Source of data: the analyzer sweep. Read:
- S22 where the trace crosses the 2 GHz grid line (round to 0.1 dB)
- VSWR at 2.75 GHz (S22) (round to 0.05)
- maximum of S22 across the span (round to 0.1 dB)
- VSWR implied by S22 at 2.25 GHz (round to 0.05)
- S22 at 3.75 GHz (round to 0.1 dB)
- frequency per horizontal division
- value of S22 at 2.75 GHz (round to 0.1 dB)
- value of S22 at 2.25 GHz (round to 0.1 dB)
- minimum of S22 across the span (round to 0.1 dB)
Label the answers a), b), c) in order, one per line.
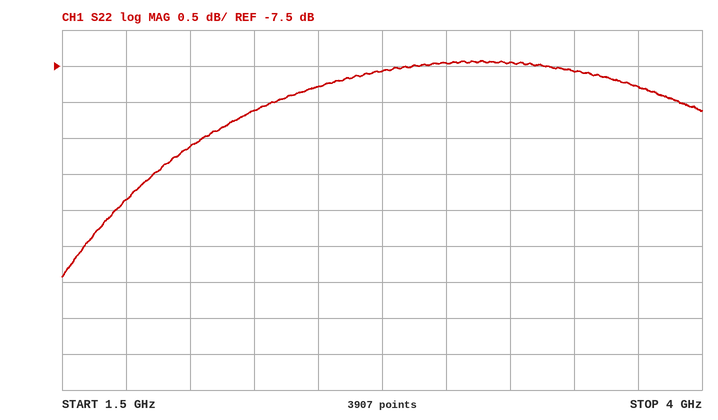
a) -8.6 dB
b) 2.45
c) -7.4 dB
d) 2.30
e) -7.8 dB
f) 250 MHz
g) -7.6 dB
h) -8.1 dB
i) -10.4 dB
